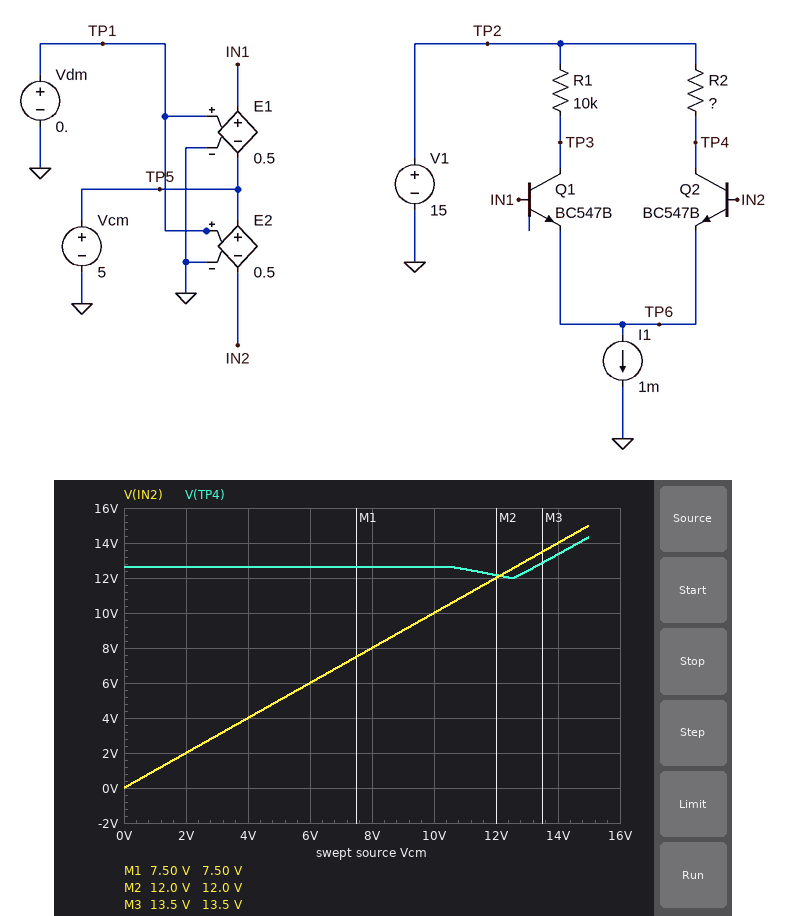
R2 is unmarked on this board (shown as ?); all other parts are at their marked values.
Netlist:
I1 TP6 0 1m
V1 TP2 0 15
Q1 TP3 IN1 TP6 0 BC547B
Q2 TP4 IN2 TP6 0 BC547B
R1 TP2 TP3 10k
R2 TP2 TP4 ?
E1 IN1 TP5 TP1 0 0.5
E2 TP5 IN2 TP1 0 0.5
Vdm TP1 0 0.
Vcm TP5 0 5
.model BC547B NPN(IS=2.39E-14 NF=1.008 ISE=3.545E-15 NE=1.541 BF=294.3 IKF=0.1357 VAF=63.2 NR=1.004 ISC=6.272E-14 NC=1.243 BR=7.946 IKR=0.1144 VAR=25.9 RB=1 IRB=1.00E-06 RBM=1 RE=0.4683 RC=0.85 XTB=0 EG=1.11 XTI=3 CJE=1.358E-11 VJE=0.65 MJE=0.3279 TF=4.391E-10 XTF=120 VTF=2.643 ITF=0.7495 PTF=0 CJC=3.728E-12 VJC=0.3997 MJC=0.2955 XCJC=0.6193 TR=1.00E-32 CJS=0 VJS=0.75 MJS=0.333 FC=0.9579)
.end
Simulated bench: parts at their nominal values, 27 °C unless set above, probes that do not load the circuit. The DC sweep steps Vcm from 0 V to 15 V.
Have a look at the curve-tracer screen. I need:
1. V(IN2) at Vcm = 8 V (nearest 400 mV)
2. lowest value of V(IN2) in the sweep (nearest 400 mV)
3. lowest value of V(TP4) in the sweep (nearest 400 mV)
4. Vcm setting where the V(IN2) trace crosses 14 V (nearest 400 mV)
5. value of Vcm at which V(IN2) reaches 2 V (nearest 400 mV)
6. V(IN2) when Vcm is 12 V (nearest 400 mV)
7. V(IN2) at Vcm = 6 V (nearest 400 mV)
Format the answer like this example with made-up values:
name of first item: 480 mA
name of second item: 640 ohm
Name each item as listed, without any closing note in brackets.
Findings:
V(IN2) at Vcm = 8 V: 8.0 V
lowest value of V(IN2) in the sweep: 0 V
lowest value of V(TP4) in the sweep: 12.0 V
Vcm setting where the V(IN2) trace crosses 14 V: 14.0 V
value of Vcm at which V(IN2) reaches 2 V: 2.0 V
V(IN2) when Vcm is 12 V: 12.0 V
V(IN2) at Vcm = 6 V: 6.0 V
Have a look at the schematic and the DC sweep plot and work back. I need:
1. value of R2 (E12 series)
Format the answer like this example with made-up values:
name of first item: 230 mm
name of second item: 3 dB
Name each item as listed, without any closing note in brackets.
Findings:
value of R2: 4.7 kΩ
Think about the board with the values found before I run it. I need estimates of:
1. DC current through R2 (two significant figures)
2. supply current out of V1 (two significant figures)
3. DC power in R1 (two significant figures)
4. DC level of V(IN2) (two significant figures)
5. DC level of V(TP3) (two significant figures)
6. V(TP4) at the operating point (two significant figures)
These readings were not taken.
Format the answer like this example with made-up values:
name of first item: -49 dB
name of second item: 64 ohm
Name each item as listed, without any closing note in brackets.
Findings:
DC current through R2: 510 µA
supply current out of V1: 1.0 mA
DC power in R1: 2.4 mW
DC level of V(IN2): 5.0 V
DC level of V(TP3): 10 V
V(TP4) at the operating point: 13 V
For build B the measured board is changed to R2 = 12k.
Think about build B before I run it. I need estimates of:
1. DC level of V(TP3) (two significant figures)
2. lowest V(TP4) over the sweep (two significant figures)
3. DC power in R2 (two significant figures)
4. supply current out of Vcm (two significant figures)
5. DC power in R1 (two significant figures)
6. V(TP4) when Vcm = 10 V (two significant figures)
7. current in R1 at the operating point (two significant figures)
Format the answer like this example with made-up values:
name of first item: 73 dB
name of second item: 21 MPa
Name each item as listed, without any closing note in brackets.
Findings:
DC level of V(TP3): 10 V
lowest V(TP4) over the sweep: 9.1 V
DC power in R2: 2.9 mW
supply current out of Vcm: 3.3 µA
DC power in R1: 2.5 mW
V(TP4) when Vcm = 10 V: 9.4 V
current in R1 at the operating point: 500 µA
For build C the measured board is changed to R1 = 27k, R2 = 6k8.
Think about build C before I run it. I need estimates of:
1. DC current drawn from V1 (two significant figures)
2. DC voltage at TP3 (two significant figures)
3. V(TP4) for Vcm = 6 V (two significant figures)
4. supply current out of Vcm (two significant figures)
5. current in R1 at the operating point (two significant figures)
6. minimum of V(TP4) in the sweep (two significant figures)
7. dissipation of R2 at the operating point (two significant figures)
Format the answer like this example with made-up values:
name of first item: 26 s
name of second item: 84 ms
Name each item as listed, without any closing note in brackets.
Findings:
DC current drawn from V1: 980 µA
DC voltage at TP3: 4.4 V
V(TP4) for Vcm = 6 V: 11 V
supply current out of Vcm: 23 µA
current in R1 at the operating point: 390 µA
minimum of V(TP4) in the sweep: 10 V
dissipation of R2 at the operating point: 2.3 mW
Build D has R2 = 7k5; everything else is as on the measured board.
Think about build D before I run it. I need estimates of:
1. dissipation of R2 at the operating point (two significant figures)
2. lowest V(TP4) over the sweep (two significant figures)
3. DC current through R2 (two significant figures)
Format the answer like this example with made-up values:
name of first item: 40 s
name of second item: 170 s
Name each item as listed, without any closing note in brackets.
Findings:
dissipation of R2 at the operating point: 1.9 mW
lowest V(TP4) over the sweep: 11 V
DC current through R2: 500 µA
